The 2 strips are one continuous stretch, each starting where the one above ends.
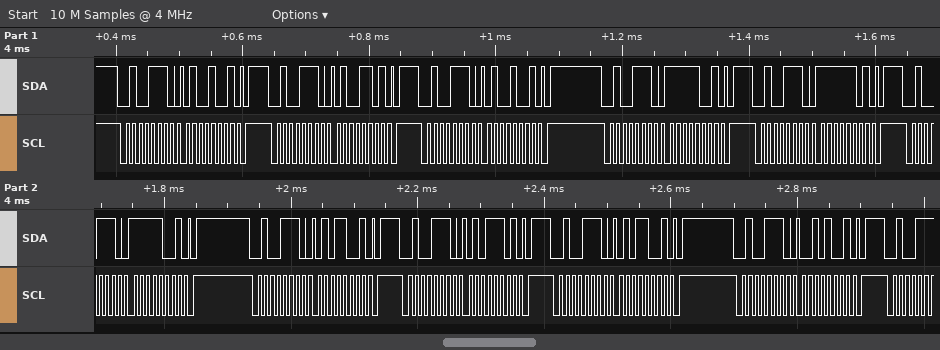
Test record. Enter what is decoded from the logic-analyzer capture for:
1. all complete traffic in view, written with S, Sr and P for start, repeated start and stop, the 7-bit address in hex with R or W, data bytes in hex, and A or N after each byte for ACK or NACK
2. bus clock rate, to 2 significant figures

S 27W A 49 A P S 27W A 4D A P S 27W A 49 A P S 27W A F9 A P S 27W A FD A P S 27W A F9 A P S 27W A 59 A P S 27W A 5D A P S 27W A 59 A P S 27W A 29 A P
100 kHz
